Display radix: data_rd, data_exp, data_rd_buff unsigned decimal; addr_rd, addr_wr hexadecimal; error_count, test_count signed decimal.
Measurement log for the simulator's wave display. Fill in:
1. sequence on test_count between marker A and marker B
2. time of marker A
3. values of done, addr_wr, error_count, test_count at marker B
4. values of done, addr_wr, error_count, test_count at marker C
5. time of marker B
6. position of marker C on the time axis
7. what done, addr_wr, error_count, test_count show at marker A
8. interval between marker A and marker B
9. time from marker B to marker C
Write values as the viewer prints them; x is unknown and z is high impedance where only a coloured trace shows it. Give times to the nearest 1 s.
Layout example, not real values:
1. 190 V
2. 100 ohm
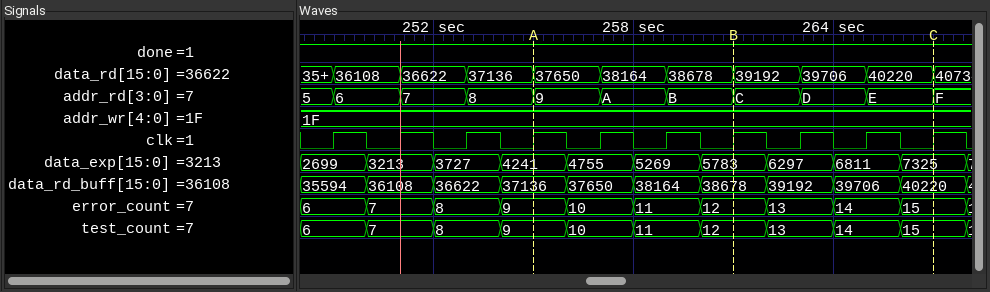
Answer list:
1. 9, 10, 11, 12
2. 255 s
3. done=1, addr_wr=1F, error_count=12, test_count=12
4. done=1, addr_wr=1F, error_count=15, test_count=15
5. 261 s
6. 267 s
7. done=1, addr_wr=1F, error_count=9, test_count=9
8. 6 s
9. 6 s
